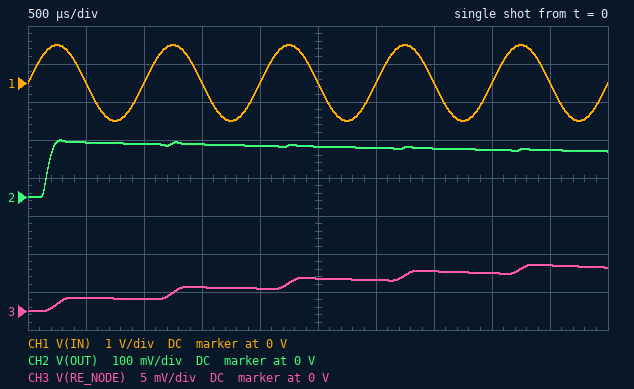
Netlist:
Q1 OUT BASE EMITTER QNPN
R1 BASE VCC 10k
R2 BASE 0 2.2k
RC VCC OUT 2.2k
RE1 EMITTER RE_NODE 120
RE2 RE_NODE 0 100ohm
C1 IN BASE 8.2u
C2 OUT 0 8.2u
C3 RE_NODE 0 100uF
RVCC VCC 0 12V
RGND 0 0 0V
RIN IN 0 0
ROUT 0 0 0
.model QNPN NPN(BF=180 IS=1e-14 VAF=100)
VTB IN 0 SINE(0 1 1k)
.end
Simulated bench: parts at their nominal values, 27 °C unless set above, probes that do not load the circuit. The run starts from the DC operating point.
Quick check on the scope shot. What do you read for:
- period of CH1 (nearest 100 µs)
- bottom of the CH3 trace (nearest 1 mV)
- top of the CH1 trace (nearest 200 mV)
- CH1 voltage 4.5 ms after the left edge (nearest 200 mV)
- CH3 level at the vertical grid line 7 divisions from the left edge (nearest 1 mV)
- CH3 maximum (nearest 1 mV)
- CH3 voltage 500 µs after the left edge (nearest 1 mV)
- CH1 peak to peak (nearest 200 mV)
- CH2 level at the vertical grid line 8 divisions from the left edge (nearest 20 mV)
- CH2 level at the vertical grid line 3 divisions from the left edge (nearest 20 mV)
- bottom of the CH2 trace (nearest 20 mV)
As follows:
1.0 ms
0 V
1.0 V
0 V
5 mV
6 mV
2 mV
2.0 V
120 mV
140 mV
0 V
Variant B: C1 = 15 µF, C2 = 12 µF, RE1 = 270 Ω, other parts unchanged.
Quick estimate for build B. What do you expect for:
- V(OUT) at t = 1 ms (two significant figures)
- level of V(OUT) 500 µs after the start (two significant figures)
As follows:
160 mV
170 mV
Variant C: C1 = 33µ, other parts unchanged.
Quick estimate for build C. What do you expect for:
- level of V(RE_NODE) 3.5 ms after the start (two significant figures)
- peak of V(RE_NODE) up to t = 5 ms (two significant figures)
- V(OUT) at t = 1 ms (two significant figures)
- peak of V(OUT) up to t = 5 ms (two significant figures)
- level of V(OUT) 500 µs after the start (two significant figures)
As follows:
10 mV
12 mV
220 mV
240 mV
230 mV
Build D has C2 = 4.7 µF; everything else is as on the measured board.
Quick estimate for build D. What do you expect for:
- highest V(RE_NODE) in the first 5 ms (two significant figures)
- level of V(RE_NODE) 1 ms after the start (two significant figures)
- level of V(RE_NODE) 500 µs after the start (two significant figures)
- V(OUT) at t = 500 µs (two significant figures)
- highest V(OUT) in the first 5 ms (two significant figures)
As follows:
7.4 mV
2.1 mV
2.2 mV
170 mV
190 mV
